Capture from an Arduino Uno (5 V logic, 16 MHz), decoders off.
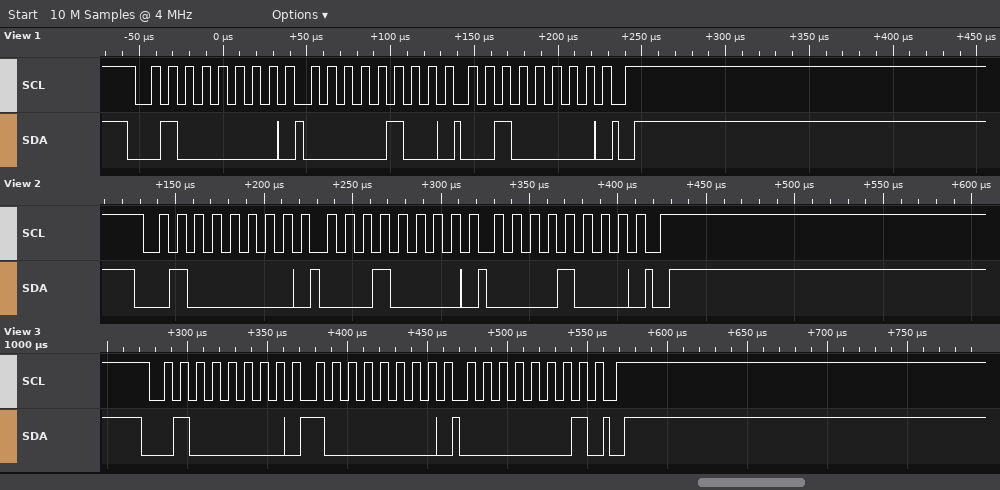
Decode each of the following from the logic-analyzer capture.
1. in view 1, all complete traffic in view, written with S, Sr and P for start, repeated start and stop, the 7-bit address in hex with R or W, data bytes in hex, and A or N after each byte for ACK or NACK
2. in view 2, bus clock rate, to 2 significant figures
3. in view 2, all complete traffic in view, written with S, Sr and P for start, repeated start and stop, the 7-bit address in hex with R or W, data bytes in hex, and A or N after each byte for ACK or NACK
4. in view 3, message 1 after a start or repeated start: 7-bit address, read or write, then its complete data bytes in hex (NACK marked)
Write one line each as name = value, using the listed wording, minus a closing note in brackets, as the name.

in view 1, all complete traffic in view, written with S, Sr and P for start, repeated start and stop, the 7-bit address in hex with R or W, data bytes in hex, and A or N after each byte for ACK or NACK = S 20W A 04 A 20 A P
in view 2, bus clock rate, to 2 significant figures = 100 kHz
in view 2, all complete traffic in view, written with S, Sr and P for start, repeated start and stop, the 7-bit address in hex with R or W, data bytes in hex, and A or N after each byte for ACK or NACK = S 20W A 10 A 08 A P
in view 3, message 1 after a start or repeated start: 7-bit address, read or write, then its complete data bytes in hex = 0x20 write: 80 01
